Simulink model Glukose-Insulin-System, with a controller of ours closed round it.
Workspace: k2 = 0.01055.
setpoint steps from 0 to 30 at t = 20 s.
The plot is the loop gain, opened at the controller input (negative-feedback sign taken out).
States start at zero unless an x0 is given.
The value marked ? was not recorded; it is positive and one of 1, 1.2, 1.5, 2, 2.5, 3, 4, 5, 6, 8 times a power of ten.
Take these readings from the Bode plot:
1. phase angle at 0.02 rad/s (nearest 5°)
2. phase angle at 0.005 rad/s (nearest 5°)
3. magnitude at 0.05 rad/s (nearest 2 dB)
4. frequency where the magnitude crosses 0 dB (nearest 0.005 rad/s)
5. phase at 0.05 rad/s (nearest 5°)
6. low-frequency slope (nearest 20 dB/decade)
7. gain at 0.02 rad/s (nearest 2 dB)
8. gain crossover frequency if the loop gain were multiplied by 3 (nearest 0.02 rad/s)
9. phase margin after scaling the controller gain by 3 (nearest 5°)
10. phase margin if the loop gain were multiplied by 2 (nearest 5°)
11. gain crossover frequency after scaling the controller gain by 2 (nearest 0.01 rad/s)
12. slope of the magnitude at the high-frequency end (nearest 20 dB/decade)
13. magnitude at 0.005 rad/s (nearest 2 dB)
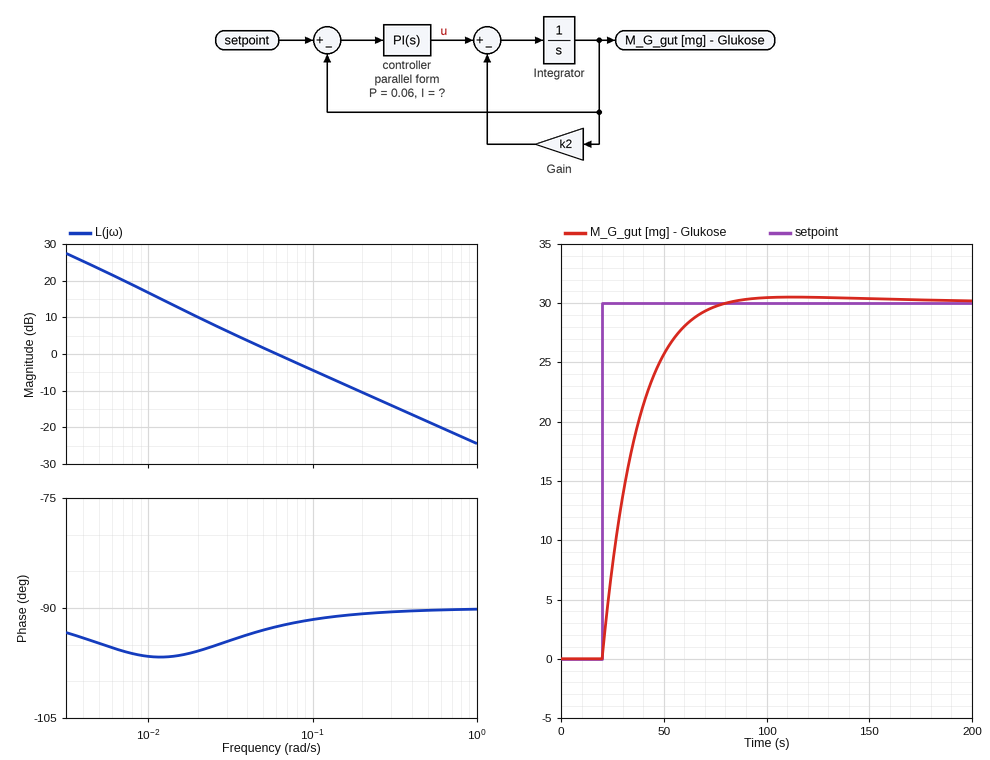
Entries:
-95°
-95°
2 dB
0.060 rad/s
-95°
-20 dB/decade
10 dB
0.18 rad/s
90°
90°
0.12 rad/s
-20 dB/decade
24 dB
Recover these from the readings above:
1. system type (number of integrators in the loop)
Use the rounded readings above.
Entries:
1
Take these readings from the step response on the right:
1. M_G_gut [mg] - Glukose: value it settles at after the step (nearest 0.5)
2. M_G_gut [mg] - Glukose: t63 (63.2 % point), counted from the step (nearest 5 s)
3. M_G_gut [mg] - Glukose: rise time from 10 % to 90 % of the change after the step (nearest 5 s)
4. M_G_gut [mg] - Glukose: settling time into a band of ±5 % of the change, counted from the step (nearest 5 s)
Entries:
30.0
15 s
35 s
45 s
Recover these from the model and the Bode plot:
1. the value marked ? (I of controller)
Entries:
0.0008
